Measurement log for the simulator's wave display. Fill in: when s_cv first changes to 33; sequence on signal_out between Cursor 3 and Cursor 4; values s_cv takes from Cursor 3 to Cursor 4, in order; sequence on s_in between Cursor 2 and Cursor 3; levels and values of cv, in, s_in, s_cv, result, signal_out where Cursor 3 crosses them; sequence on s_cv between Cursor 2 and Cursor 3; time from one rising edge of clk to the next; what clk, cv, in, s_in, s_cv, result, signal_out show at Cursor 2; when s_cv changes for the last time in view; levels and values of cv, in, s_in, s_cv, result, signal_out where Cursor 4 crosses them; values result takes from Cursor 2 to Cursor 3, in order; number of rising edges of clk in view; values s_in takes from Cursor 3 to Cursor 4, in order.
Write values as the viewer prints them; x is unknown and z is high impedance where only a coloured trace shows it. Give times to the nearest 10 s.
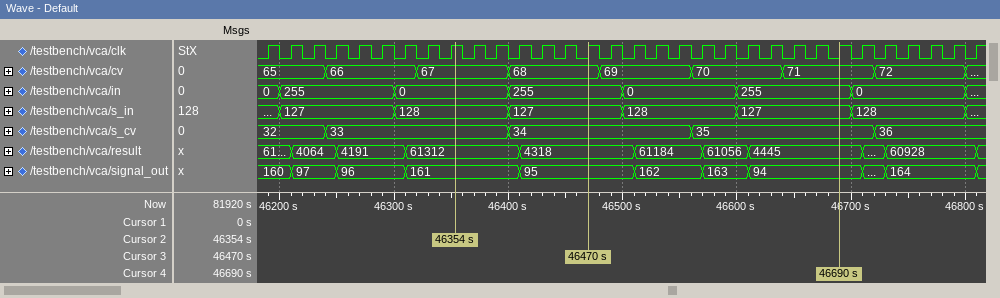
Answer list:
46240 s
95, 162, 163, 94
34, 35
128, 127
cv=68, in=255, s_in=127, s_cv=34, result=4318, signal_out=95
33, 34
20 s
clk=1, cv=67, in=0, s_in=128, s_cv=33, result=61312, signal_out=161
46720 s
cv=71, in=255, s_in=127, s_cv=35, result=4445, signal_out=94
61312, 4318
32
127, 128, 127
